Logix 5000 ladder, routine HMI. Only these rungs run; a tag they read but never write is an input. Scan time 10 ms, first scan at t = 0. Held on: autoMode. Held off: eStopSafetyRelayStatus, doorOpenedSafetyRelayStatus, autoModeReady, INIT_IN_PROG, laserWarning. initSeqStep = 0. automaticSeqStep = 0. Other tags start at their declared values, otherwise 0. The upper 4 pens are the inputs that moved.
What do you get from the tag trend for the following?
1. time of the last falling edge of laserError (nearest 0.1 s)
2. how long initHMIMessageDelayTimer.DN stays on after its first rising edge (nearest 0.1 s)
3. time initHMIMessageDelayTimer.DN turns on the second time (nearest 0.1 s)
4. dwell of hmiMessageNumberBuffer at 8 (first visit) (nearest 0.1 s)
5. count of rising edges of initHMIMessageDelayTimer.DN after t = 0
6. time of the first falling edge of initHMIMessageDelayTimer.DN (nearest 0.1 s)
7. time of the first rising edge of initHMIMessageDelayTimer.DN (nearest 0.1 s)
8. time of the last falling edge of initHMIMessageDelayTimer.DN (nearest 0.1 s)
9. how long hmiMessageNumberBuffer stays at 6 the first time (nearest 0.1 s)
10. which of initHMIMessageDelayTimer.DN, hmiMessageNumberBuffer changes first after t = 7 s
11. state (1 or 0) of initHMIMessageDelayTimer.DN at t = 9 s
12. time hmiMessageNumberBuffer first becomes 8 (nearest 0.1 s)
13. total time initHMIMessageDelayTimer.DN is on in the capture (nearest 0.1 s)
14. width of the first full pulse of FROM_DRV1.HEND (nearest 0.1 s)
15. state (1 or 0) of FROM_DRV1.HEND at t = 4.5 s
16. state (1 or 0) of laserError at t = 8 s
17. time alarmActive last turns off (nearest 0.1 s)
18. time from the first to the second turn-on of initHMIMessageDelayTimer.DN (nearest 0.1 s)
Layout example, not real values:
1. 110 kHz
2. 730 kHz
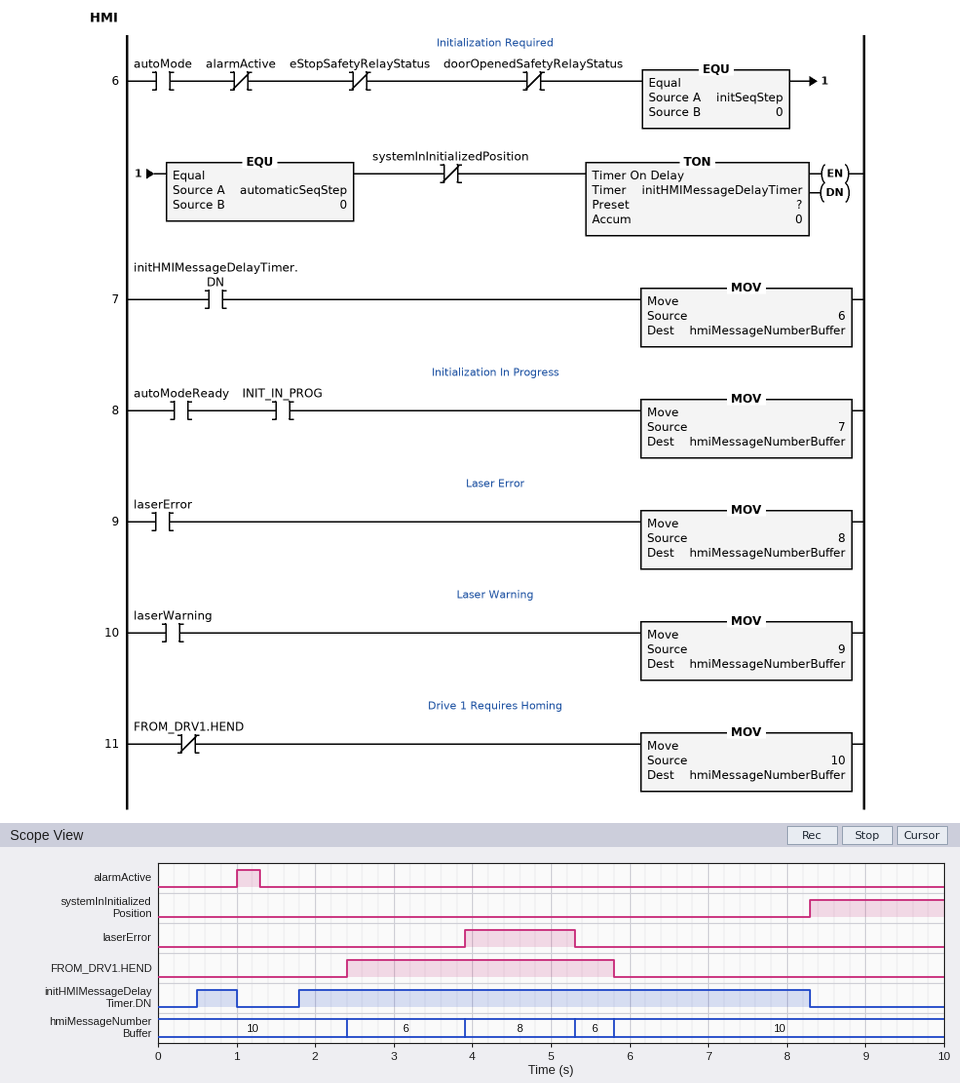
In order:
1. 5.3 s
2. 0.5 s
3. 1.8 s
4. 1.4 s
5. 2
6. 1.0 s
7. 0.5 s
8. 8.3 s
9. 1.5 s
10. initHMIMessageDelayTimer.DN
11. 0
12. 3.9 s
13. 7.0 s
14. 3.4 s
15. 1
16. 0
17. 1.3 s
18. 1.3 s
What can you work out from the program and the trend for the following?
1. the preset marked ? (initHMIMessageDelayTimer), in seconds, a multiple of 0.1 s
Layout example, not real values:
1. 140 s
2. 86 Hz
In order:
1. 0.5 s
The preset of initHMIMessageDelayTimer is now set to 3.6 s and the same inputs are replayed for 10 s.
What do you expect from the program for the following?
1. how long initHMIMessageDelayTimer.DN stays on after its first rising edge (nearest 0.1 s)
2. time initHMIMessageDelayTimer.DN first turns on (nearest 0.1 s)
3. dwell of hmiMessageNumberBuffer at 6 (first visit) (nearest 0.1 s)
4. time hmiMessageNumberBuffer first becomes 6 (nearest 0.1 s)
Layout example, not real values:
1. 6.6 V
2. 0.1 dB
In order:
1. 3.4 s
2. 4.9 s
3. 0.5 s
4. 5.3 s
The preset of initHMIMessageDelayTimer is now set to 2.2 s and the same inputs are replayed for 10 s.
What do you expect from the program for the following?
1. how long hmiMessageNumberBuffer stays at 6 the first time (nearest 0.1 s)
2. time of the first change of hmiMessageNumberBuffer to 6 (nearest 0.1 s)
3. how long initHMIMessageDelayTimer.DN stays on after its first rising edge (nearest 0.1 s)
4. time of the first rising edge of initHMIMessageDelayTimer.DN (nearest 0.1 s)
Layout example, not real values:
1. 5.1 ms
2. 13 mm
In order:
1. 0.4 s
2. 3.5 s
3. 4.8 s
4. 3.5 s
